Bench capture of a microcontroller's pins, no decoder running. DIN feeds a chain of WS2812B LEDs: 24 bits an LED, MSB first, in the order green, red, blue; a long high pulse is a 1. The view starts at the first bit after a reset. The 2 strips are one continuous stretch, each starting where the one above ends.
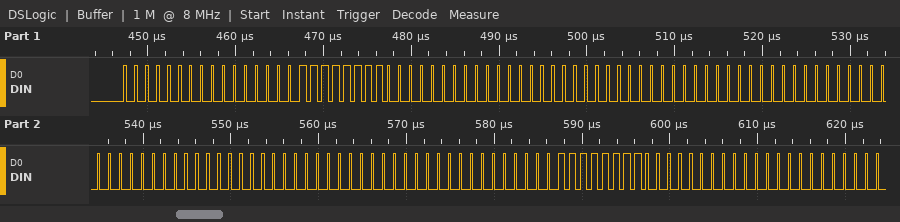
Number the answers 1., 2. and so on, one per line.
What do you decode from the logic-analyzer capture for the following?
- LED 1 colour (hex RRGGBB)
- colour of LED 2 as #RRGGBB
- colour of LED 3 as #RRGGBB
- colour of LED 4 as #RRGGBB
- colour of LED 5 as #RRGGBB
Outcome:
1. #0000FF
2. #000000
3. #000000
4. #000000
5. #0000FF
